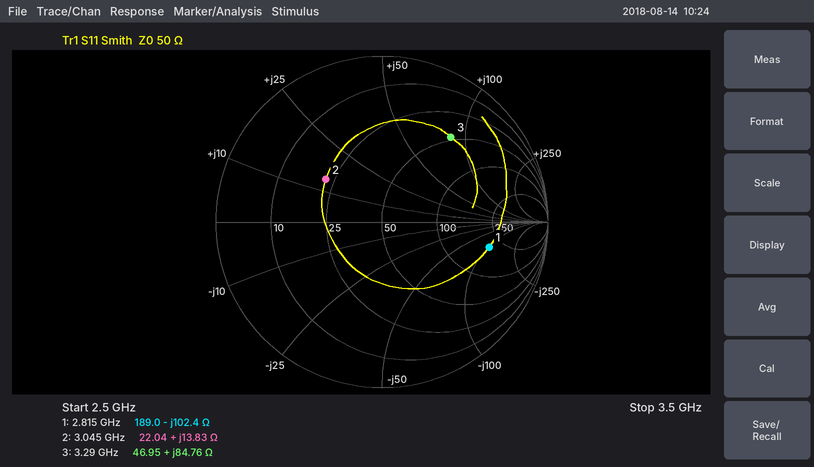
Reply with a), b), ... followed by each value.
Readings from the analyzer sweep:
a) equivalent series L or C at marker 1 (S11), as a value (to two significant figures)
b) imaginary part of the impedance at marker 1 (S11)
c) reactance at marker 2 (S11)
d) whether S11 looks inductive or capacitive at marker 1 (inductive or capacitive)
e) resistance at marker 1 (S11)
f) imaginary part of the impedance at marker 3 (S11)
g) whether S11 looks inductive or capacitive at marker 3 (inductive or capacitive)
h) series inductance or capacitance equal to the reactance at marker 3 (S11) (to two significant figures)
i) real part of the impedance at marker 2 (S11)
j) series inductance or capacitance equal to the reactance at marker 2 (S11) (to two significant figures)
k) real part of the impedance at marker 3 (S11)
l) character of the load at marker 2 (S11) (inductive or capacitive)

a) 550 fF
b) -102.4 Ω
c) +13.83 Ω
d) capacitive
e) 189.0 Ω
f) +84.76 Ω
g) inductive
h) 4.1 nH
i) 22.04 Ω
j) 720 pH
k) 46.95 Ω
l) inductive
